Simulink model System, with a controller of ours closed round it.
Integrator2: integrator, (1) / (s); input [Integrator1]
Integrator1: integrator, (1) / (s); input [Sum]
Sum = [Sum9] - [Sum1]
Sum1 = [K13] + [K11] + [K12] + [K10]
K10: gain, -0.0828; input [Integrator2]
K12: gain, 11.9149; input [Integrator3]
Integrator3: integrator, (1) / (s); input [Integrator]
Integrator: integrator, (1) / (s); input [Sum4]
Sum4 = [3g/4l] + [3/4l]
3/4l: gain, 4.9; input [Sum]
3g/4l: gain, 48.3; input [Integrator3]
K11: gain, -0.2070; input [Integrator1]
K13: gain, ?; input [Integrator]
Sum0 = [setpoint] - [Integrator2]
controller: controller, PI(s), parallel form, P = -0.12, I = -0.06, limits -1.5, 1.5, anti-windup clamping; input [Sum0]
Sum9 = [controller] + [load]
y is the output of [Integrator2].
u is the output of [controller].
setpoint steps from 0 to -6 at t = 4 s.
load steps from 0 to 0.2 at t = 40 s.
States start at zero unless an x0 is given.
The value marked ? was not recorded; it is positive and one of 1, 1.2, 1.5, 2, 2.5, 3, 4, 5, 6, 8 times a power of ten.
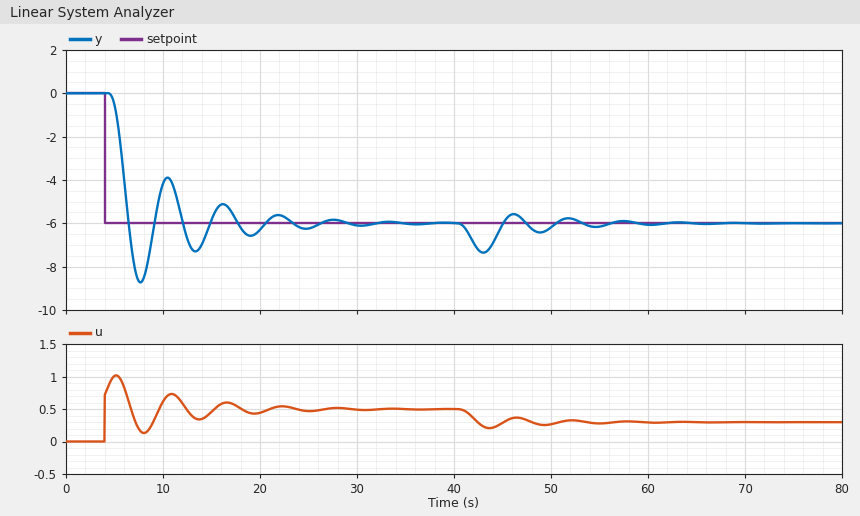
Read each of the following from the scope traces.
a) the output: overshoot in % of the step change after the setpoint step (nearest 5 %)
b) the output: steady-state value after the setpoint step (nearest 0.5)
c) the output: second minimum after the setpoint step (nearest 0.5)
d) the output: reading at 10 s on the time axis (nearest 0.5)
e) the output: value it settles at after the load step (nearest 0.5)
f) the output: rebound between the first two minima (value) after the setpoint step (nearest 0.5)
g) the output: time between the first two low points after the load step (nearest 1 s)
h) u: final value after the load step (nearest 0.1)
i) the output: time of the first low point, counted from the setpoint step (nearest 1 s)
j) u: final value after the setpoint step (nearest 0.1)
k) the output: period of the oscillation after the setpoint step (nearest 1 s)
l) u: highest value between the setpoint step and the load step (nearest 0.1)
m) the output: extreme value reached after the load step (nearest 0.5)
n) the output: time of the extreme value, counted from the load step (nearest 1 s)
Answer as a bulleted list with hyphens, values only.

- 45 %
- -6.0
- -7.5
- -4.0
- -6.0
- -4.0
- 6 s
- 0.3
- 4 s
- 0.5
- 6 s
- 1.0
- -7.5
- 3 s
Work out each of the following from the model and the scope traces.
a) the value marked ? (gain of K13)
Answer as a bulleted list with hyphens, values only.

- 1
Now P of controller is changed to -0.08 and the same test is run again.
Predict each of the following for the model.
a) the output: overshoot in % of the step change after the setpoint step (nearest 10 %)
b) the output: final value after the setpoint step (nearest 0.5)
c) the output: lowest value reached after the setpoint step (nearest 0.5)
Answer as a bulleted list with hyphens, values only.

- 40 %
- -6.0
- -8.5
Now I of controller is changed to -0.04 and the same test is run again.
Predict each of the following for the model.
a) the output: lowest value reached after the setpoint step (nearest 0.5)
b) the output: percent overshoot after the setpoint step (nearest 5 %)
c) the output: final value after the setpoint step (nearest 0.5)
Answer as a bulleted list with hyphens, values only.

- -7.5
- 25 %
- -6.0
